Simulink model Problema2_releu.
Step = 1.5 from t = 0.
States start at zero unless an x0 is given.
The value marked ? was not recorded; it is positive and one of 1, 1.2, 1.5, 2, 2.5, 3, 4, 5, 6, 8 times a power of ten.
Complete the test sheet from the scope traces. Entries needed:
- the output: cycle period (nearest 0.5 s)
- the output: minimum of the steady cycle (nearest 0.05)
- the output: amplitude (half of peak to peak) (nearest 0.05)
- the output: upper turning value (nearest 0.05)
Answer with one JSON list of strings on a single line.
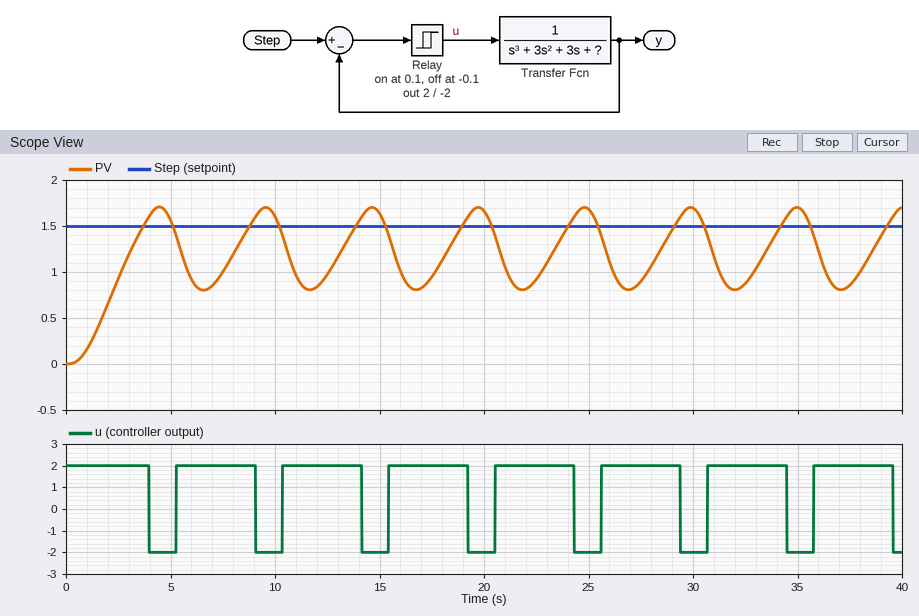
["5.0 s", "0.80", "0.45", "1.70"]
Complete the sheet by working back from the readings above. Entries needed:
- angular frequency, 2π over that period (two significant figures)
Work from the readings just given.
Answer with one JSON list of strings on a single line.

["1.3 rad/s"]
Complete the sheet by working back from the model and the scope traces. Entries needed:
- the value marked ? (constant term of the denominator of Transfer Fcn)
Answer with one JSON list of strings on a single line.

["0.8"]
